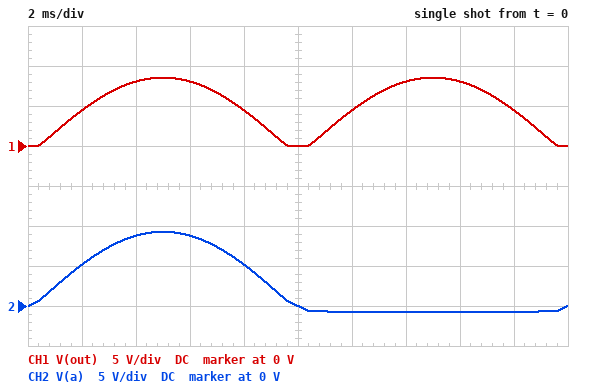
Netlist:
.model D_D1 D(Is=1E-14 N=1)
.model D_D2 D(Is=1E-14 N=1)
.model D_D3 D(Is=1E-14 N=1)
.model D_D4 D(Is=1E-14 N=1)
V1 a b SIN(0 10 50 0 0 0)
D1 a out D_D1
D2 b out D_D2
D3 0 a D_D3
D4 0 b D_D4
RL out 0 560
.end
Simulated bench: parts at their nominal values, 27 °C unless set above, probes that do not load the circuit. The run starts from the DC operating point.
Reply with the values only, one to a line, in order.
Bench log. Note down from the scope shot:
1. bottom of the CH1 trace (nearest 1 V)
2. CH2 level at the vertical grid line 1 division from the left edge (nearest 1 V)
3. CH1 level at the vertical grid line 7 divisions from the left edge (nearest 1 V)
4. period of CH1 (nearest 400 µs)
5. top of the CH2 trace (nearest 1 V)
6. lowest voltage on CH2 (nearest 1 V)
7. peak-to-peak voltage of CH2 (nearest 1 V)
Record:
0 V
5 V
8 V
10.0 ms
9 V
-1 V
10 V
